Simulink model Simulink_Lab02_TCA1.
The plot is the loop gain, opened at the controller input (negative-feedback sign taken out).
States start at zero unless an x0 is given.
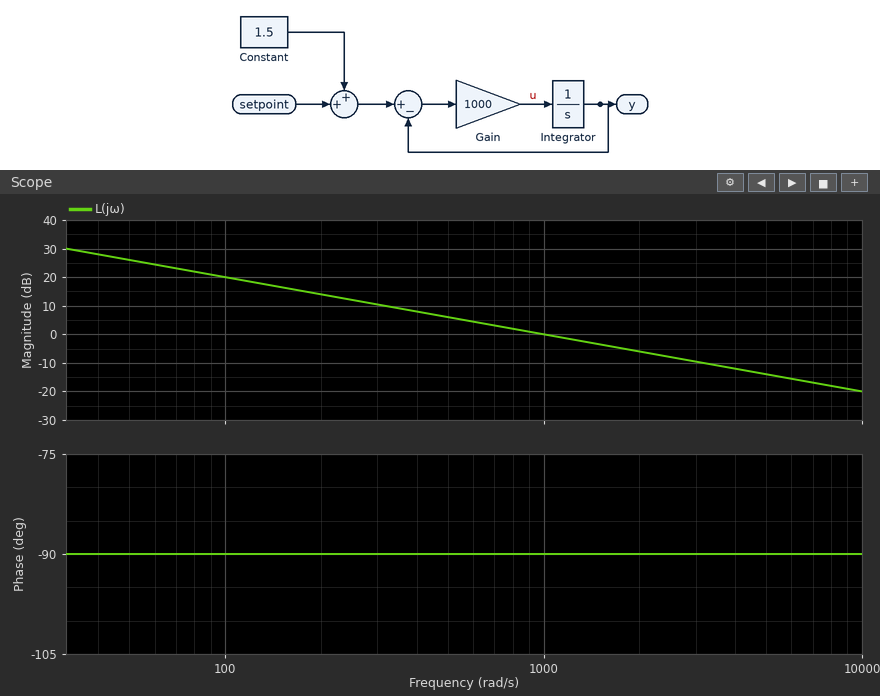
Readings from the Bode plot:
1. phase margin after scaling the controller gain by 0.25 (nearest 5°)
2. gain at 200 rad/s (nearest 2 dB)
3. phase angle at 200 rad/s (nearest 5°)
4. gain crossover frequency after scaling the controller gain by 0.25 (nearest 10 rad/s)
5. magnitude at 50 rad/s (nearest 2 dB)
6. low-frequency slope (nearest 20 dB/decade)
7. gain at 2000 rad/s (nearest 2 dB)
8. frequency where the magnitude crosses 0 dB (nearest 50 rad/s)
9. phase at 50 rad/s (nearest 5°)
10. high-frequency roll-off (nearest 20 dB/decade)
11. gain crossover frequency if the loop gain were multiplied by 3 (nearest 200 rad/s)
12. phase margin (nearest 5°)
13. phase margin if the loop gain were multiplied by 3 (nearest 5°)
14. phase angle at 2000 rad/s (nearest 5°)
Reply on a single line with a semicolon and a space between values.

90°; 14 dB; -90°; 250 rad/s; 26 dB; -20 dB/decade; -6 dB; 1000 rad/s; -90°; -20 dB/decade; 3000 rad/s; 90°; 90°; -90°
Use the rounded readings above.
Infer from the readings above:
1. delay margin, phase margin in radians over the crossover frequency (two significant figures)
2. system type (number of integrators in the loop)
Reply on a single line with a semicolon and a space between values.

0.0016 s; 1
